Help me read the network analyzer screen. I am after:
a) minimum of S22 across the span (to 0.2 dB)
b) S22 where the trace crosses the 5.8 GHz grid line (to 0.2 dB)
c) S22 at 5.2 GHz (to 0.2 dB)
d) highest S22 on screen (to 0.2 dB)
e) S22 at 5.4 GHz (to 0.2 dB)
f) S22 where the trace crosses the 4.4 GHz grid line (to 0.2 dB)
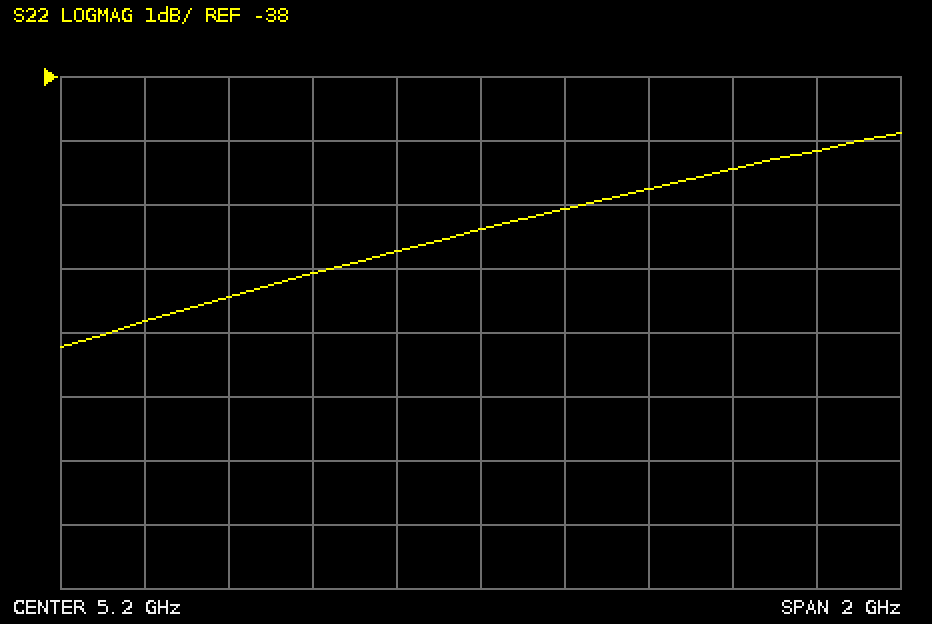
-42.2 dB
-39.4 dB
-40.4 dB
-38.8 dB
-40.0 dB
-41.8 dB
